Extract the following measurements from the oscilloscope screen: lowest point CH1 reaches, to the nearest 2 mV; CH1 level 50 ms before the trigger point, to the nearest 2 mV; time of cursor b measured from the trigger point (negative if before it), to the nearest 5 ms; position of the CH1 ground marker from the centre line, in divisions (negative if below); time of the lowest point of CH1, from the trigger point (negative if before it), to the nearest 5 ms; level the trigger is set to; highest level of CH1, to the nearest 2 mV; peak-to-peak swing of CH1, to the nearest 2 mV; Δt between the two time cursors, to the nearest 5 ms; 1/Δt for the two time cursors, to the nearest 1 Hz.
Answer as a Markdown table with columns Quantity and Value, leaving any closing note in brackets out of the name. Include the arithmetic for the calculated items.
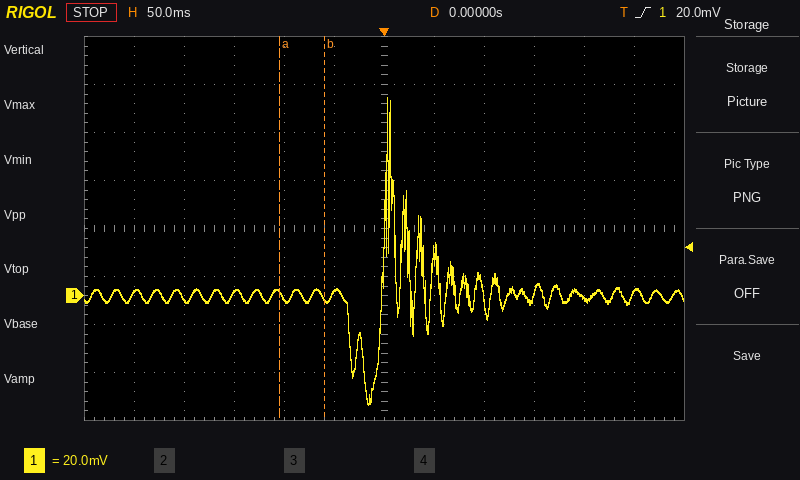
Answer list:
| Quantity | Value |
|---|---|
| lowest point CH1 reaches, to the nearest 2 mV | -46 mV |
| CH1 level 50 ms before the trigger point, to the nearest 2 mV | 2 mV |
| time of cursor b measured from the trigger point (negative if before it), to the nearest 5 ms | -60 ms |
| position of the CH1 ground marker from the centre line, in divisions | -1.4 div |
| time of the lowest point of CH1, from the trigger point (negative if before it), to the nearest 5 ms | -15 ms |
| level the trigger is set to | 20.0 mV |
| highest level of CH1, to the nearest 2 mV | 82 mV |
| peak-to-peak swing of CH1, to the nearest 2 mV | 82 mV − (-46 mV) = 128 mV |
| Δt between the two time cursors, to the nearest 5 ms | 45 ms |
| 1/Δt for the two time cursors, to the nearest 1 Hz | 1 / 45 ms ≈ 22 Hz |
